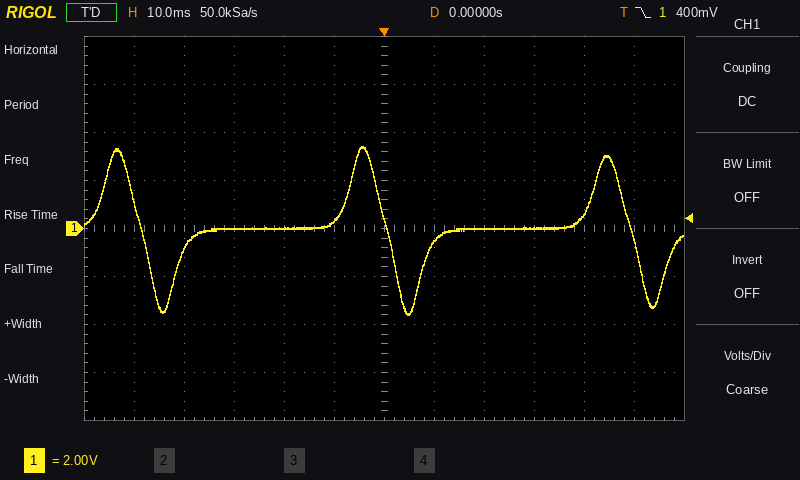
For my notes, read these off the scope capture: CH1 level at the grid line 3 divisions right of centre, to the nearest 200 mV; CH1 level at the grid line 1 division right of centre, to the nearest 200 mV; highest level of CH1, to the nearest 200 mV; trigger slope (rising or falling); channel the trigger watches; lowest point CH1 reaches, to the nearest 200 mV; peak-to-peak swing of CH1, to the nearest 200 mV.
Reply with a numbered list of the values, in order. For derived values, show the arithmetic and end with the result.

1. 0.0 V
2. -600 mV
3. 3.4 V
4. falling
5. CH1
6. -3.6 V
7. 3.4 V − (-3.6 V) = 7.0 V
